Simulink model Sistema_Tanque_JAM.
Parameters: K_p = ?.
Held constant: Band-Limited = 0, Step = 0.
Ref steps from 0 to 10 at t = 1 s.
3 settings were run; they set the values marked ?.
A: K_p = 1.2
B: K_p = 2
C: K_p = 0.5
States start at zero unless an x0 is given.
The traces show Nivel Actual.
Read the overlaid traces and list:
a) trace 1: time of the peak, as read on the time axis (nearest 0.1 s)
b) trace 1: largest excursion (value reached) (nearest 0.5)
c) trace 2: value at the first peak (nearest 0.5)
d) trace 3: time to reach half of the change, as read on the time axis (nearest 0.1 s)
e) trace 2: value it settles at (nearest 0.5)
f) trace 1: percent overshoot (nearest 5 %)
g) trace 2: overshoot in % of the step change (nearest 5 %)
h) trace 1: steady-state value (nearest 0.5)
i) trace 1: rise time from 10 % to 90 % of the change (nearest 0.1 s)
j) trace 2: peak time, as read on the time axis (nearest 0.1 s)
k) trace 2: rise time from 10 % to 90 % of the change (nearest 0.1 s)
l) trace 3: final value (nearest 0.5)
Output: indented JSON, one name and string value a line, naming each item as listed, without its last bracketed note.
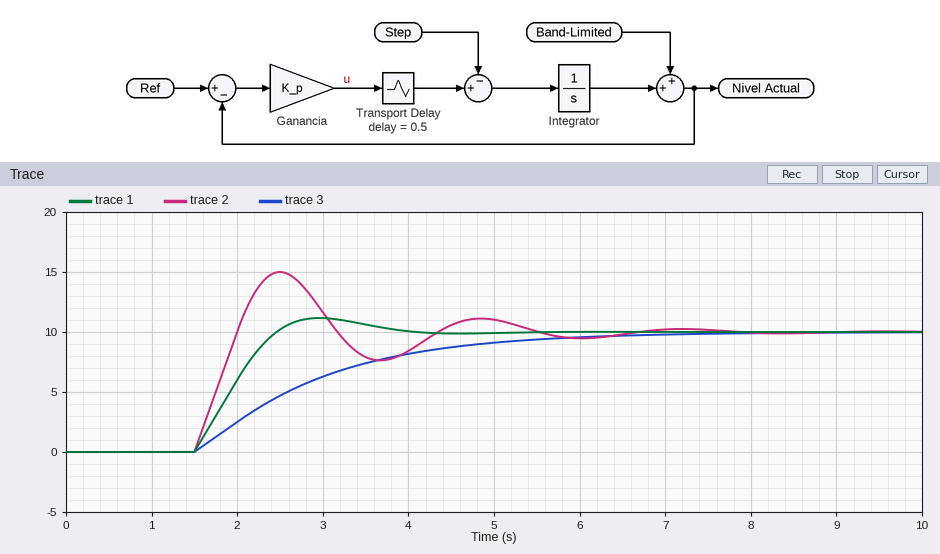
{
  "trace 1: time of the peak, as read on the time axis": "3.0 s",
  "trace 1: largest excursion (value reached)": "11.0",
  "trace 2: value at the first peak": "15.0",
  "trace 3: time to reach half of the change, as read on the time axis": "2.6 s",
  "trace 2: value it settles at": "10.0",
  "trace 1: percent overshoot": "10 %",
  "trace 2: overshoot in % of the step change": "50 %",
  "trace 1: steady-state value": "10.0",
  "trace 1: rise time from 10 % to 90 % of the change": "0.7 s",
  "trace 2: peak time, as read on the time axis": "2.5 s",
  "trace 2: rise time from 10 % to 90 % of the change": "0.4 s",
  "trace 3: final value": "10.0"
}
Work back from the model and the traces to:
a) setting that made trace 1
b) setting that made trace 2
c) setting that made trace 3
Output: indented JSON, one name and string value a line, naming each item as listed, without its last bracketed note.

{
  "setting that made trace 1": "A",
  "setting that made trace 2": "B",
  "setting that made trace 3": "C"
}
